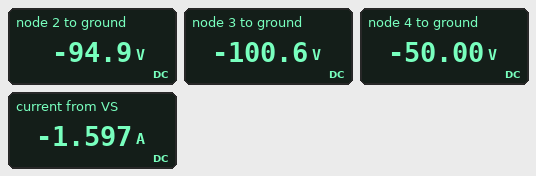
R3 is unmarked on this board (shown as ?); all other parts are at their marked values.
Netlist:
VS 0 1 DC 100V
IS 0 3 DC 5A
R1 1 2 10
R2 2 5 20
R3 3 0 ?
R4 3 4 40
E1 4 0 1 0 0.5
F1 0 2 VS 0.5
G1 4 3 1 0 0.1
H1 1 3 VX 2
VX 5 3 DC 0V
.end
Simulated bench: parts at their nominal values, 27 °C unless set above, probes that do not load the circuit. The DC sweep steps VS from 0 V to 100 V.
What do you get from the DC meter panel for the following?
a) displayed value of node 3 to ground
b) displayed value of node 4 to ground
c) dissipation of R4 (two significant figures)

-100.6 V
-50.00 V
64 W
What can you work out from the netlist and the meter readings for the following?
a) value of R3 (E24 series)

75 Ω
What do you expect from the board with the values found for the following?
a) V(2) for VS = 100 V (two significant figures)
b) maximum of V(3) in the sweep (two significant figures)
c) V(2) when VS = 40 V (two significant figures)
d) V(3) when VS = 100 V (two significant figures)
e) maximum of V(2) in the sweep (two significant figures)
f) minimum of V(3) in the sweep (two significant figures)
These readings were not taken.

-95 V
1.2 V
-44 V
-100 V
-11 V
-100 V
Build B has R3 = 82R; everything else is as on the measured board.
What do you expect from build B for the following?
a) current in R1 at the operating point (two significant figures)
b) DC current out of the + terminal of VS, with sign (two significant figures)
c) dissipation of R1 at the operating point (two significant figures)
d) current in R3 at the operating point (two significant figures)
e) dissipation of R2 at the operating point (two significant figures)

540 mA
-1.7 A
2.9 W
1.2 A
1.8 W
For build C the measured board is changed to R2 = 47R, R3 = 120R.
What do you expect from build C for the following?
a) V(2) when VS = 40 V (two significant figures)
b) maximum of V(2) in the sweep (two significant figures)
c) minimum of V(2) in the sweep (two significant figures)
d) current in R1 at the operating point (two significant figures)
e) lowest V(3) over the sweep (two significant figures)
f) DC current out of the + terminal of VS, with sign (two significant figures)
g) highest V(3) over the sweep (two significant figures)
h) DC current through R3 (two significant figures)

-45 V
-14 V
-92 V
790 mA
-100 V
-1.9 A
600 mV
840 mA
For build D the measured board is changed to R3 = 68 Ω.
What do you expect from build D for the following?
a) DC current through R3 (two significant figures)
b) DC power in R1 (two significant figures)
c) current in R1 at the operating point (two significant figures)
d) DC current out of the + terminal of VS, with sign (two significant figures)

1.5 A
2.3 W
480 mA
-1.5 A
